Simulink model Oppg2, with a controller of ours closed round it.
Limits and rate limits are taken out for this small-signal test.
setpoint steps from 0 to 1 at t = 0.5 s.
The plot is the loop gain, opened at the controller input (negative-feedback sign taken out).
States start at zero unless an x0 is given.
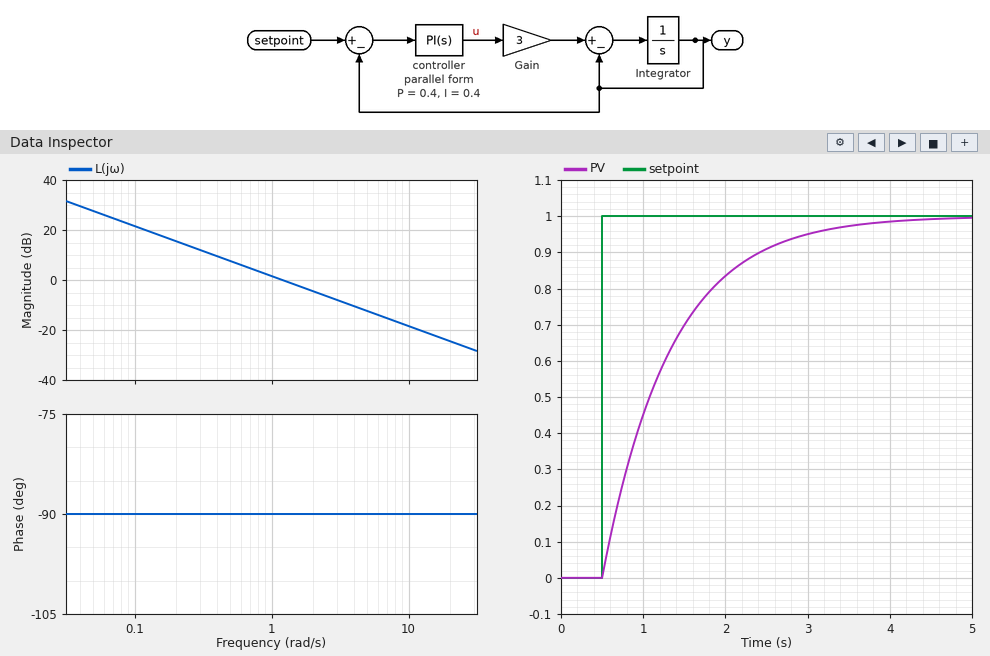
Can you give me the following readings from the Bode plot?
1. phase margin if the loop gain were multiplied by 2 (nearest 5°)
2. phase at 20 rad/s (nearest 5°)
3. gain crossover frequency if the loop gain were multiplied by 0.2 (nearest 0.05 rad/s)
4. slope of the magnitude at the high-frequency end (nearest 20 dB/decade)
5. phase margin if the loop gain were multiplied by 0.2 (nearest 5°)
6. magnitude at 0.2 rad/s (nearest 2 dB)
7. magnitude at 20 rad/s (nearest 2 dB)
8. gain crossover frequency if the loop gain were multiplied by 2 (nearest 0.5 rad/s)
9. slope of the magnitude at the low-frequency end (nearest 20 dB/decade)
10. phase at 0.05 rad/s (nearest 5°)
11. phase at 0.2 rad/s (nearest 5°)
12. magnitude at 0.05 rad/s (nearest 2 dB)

90°
-90°
0.25 rad/s
-20 dB/decade
90°
16 dB
-24 dB
2.5 rad/s
-20 dB/decade
-90°
-90°
28 dB
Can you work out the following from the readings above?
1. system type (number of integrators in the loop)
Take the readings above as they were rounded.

1
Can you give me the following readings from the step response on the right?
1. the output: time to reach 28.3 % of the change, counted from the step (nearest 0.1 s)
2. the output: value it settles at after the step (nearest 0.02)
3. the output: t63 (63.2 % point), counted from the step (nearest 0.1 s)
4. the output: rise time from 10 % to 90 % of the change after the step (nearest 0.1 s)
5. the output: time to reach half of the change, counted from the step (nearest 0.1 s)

0.3 s
1.00
0.8 s
1.8 s
0.6 s
